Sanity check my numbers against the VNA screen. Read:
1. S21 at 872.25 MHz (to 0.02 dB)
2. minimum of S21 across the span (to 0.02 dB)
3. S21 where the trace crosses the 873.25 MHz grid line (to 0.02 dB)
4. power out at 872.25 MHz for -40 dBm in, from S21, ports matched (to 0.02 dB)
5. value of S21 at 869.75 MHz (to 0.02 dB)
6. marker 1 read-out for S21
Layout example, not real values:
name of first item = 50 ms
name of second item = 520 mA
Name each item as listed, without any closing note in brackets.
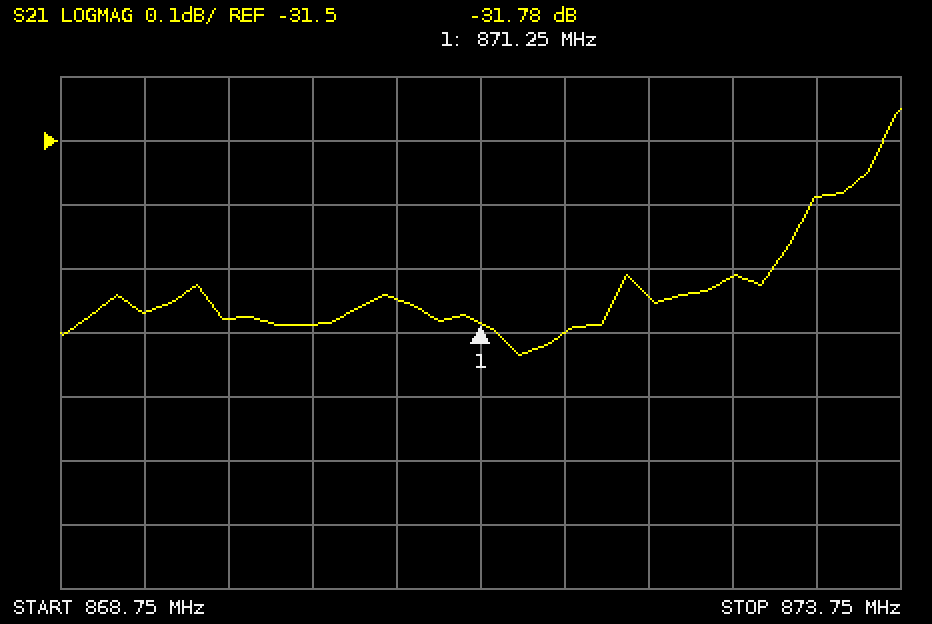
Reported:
S21 at 872.25 MHz = -31.74 dB
minimum of S21 across the span = -31.84 dB
S21 where the trace crosses the 873.25 MHz grid line = -31.58 dB
power out at 872.25 MHz for -40 dBm in, from S21, ports matched = -71.74 dBm
value of S21 at 869.75 MHz = -31.78 dB
marker 1 read-out for S21 = -31.78 dB
